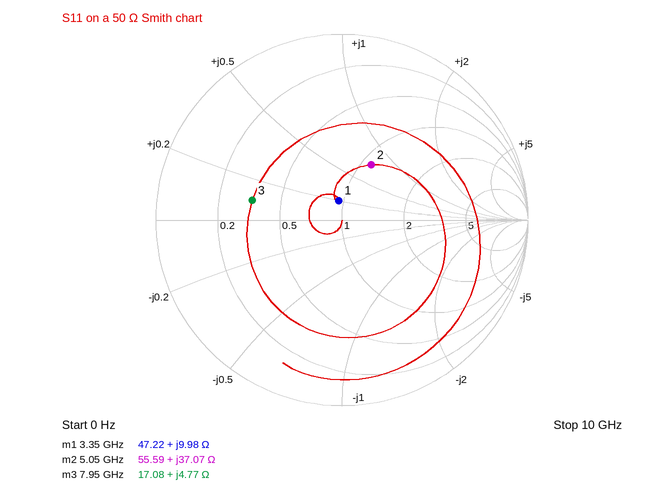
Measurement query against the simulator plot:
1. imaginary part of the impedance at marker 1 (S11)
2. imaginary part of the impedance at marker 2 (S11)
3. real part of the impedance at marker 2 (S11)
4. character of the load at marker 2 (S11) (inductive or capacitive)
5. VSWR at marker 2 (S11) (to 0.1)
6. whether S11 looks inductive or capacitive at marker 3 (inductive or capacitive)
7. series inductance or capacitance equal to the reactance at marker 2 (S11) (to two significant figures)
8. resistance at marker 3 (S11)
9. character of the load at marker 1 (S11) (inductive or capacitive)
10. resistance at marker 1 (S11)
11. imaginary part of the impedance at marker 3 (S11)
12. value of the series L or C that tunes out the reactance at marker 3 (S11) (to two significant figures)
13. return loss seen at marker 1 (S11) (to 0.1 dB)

+9.98 Ω
+37.07 Ω
55.59 Ω
inductive
2.0
inductive
1.2 nH
17.08 Ω
inductive
47.22 Ω
+4.77 Ω
4.2 pF
19.5 dB
